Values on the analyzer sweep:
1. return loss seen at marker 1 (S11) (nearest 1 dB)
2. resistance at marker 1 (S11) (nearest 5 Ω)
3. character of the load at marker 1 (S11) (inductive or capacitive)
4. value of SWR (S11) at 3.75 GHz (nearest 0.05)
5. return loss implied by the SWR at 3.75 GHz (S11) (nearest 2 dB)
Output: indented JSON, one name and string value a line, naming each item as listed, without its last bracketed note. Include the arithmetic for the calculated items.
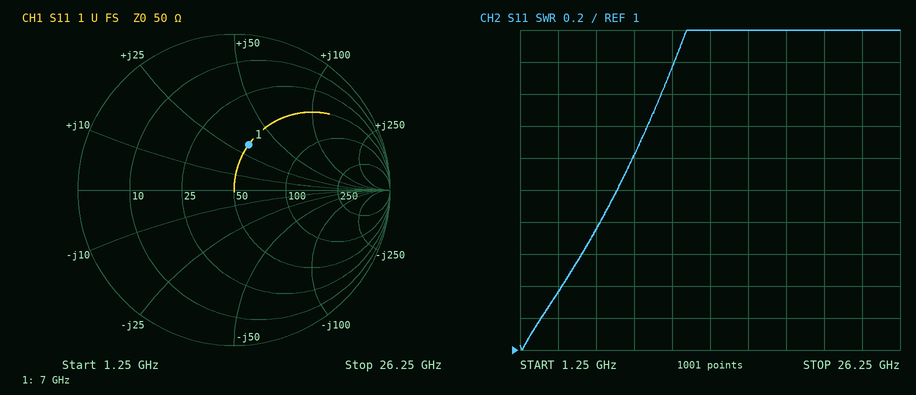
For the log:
{
  "return loss seen at marker 1 (S11)": "10 dB",
  "resistance at marker 1 (S11)": "50 Ω",
  "character of the load at marker 1 (S11)": "inductive",
  "value of SWR (S11) at 3.75 GHz": "1.35",
  "return loss implied by the SWR at 3.75 GHz (S11)": "−20 log10((1.35 − 1)/(1.35 + 1)) ≈ 16 dB"
}
